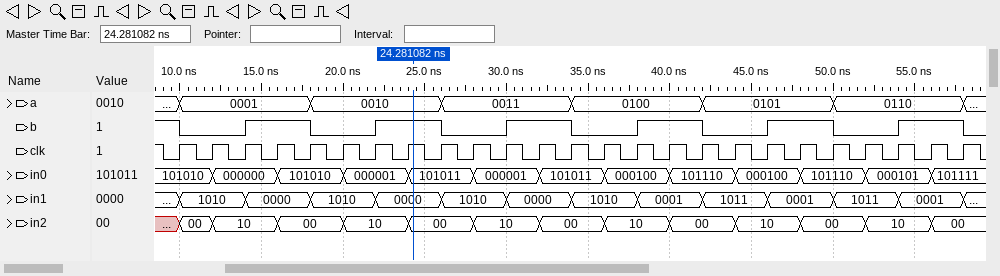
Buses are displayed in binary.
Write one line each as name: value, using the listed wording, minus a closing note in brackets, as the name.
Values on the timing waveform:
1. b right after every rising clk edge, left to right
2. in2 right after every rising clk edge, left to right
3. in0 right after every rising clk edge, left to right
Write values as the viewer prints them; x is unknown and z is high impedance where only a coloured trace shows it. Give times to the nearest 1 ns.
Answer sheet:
b right after every rising clk edge, left to right: 0 0 1 1 0 0 1 1 0 0 1 1 0 0 1 1 0 0 1 1 0 0 1 1 0
in2 right after every rising clk edge, left to right: 00, 10, 10, 00, 00, 10, 10, 00, 00, 10, 10, 00, 00, 10, 10, 00, 00, 10, 10, 00, 00, 10, 10, 00, 00
in0 right after every rising clk edge, left to right: 101010, 000000, 000000, 101010, 101010, 000001, 000001, 101011, 101011, 000001, 000001, 101011, 101011, 000100, 000100, 101110, 101110, 000100, 000100, 101110, 101110, 000101, 000101, 101111, 101111
